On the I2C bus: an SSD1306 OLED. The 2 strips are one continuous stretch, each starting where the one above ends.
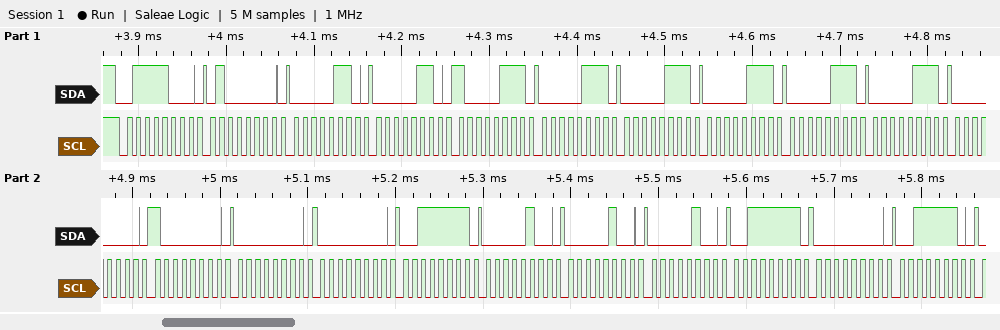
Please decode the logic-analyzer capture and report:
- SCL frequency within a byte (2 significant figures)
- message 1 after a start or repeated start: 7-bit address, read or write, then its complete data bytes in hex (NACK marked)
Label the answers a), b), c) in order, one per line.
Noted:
a) 100 kHz
b) 0x3C write: 40 06 06 87 07 07 07 07 07 00 80 00 00 3F 04 04 04 3F 00 3E
